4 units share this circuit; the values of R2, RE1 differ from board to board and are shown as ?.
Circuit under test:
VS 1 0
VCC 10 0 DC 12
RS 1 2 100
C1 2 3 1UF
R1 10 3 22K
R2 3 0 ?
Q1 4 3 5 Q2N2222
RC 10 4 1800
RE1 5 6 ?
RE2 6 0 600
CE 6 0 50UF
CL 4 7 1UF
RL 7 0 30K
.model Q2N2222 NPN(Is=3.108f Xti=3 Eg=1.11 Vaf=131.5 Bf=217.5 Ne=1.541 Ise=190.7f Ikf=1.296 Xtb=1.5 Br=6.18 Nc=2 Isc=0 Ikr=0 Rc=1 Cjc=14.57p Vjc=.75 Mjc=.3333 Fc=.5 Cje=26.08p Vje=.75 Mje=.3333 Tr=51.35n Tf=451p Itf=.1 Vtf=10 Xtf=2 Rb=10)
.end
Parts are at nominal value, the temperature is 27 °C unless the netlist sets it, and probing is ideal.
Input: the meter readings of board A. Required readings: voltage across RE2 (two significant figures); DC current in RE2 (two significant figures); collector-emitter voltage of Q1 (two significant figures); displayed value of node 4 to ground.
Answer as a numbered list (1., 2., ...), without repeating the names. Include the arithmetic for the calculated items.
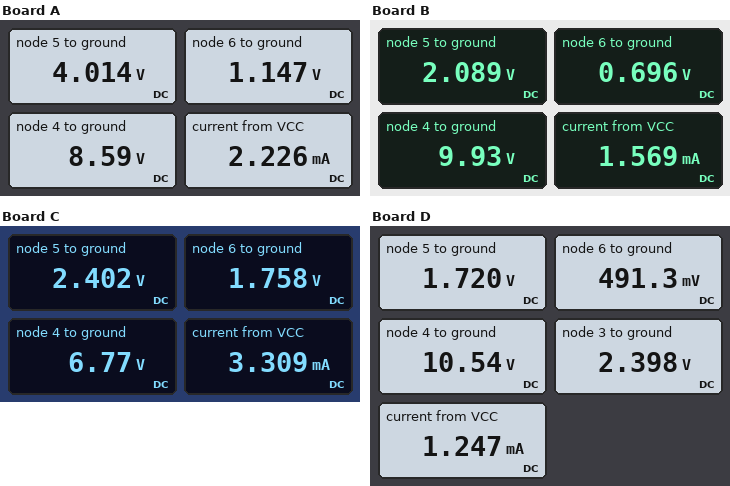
1. 1.147 V = 1.1 V
2. (1.147 V) / 600 Ω = 1.9 mA
3. 8.59 V - 4.014 V = 4.6 V
4. 8.59 V
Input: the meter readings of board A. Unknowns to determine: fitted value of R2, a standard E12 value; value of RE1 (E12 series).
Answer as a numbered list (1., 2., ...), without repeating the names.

1. 15 kΩ
2. 1.5 kΩ
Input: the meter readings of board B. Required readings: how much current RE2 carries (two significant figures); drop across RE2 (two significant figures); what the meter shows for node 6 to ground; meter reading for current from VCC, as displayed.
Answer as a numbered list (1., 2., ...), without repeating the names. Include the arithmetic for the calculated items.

1. (696 mV) / 600 Ω = 1.2 mA
2. 696 mV = 700 mV
3. 0.696 V
4. 1.569 mA
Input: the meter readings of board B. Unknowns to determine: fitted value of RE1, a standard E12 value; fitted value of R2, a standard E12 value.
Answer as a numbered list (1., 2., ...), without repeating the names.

1. 1.2 kΩ
2. 6.8 kΩ
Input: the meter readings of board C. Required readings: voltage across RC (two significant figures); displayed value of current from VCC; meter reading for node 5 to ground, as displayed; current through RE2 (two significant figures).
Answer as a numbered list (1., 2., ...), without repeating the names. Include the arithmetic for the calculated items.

1. 12 V - 6.77 V = 5.2 V
2. 3.309 mA
3. 2.402 V
4. (1.758 V) / 600 Ω = 2.9 mA
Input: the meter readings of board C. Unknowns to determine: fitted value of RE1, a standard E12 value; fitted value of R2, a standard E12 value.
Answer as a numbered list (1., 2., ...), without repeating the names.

1. 220 Ω
2. 8.2 kΩ
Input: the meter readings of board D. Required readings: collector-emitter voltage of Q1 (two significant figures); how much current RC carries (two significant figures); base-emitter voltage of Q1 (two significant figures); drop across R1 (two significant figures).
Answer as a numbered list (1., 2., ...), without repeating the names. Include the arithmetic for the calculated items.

1. 10.54 V - 1.72 V = 8.8 V
2. (12 V - 10.54 V) / 1.8 kΩ = 810 µA
3. 2.398 V - 1.72 V = 680 mV
4. 12 V - 2.398 V = 9.6 V
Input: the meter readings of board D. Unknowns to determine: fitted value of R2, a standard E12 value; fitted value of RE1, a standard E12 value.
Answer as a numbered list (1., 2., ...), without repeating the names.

1. 5.6 kΩ
2. 1.5 kΩ
